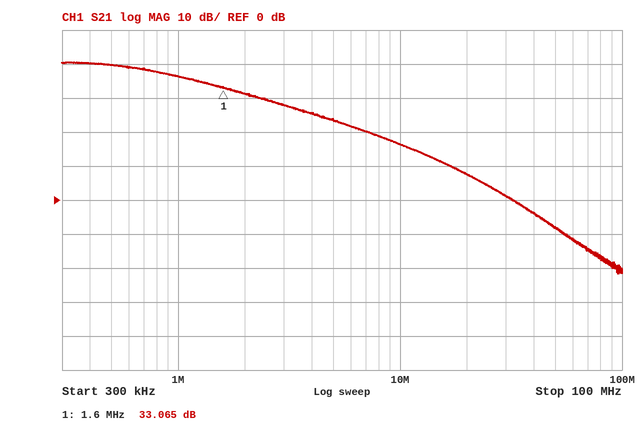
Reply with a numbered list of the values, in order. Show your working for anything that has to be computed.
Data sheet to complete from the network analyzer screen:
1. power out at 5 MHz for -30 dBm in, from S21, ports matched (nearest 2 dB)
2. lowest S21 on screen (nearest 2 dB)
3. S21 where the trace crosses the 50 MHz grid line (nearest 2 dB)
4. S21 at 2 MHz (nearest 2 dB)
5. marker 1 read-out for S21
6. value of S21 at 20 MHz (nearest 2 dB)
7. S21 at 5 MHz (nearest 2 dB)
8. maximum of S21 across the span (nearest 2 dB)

1. -30 dBm + (24 dB) = -6 dBm
2. -22 dB
3. -8 dB
4. 32 dB
5. 33.065 dB
6. 8 dB
7. 24 dB
8. 40 dB
